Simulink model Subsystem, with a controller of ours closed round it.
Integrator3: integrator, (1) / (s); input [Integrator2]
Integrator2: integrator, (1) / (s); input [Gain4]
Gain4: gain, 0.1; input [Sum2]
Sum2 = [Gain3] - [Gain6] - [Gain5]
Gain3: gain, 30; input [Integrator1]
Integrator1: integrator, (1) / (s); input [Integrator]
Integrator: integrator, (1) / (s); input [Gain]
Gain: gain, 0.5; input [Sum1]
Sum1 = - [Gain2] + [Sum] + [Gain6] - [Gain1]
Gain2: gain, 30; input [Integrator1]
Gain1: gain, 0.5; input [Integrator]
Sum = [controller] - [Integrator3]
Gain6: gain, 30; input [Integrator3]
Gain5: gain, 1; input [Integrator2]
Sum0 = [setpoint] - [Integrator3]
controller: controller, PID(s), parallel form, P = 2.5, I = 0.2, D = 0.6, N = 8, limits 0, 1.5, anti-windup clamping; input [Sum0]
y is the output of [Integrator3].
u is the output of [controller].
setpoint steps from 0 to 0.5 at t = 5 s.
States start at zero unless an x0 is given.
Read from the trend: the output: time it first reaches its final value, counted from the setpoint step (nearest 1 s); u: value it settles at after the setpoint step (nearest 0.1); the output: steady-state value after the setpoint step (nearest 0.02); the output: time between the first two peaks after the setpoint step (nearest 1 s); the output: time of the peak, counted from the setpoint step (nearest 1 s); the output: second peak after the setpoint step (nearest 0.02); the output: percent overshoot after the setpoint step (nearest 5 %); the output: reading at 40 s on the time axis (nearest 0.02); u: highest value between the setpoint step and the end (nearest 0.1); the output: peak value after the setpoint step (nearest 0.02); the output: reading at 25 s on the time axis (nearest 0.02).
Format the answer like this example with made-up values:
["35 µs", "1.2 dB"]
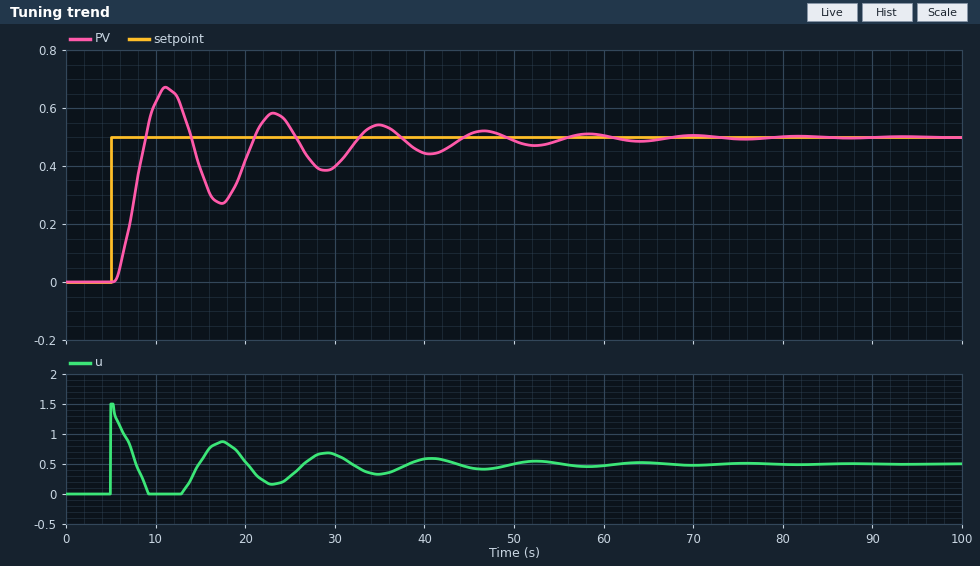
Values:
["4 s", "0.5", "0.50", "12 s", "6 s", "0.58", "35 %", "0.44", "1.5", "0.68", "0.54"]
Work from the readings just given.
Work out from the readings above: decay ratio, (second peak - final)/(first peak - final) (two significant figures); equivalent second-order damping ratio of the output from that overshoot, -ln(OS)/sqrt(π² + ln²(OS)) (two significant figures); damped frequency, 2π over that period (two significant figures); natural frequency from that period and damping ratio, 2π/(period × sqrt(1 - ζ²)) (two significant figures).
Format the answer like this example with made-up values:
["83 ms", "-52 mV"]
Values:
["0.44", "0.32", "0.52 rad/s", "0.55 rad/s"]
